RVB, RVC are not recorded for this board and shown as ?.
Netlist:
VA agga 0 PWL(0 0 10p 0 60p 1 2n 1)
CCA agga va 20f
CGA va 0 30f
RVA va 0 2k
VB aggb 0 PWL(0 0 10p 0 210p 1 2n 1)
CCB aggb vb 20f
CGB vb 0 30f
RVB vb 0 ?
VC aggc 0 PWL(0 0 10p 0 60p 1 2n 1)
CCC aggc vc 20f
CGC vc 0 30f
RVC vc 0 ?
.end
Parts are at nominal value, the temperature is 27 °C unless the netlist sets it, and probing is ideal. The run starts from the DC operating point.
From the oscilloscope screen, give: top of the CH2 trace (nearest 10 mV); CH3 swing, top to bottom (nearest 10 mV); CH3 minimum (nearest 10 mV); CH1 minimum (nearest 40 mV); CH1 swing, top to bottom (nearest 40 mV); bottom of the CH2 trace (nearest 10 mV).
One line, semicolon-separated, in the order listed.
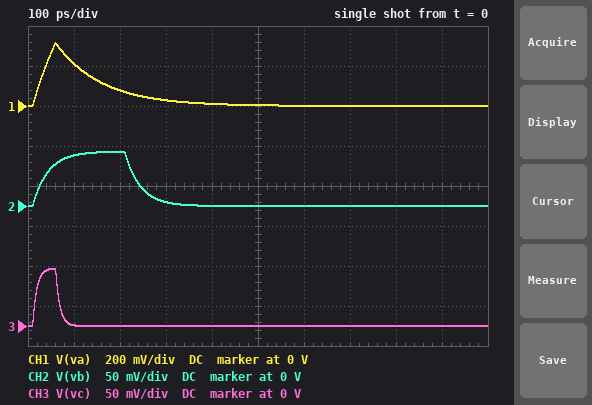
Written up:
70 mV; 70 mV; 0 V; 0 V; 320 mV; 0 V
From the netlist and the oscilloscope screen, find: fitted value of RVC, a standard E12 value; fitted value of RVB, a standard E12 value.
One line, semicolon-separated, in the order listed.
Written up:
180 Ω; 680 Ω
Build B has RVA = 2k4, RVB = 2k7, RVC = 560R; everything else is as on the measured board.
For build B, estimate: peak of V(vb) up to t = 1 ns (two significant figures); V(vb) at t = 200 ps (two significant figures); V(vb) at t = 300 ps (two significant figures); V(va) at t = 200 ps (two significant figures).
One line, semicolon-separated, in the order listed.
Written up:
210 mV; 200 mV; 110 mV; 100 mV
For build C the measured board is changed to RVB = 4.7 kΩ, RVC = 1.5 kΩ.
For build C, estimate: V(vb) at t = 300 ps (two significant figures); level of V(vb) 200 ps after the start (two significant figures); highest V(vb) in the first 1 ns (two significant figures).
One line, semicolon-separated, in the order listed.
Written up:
180 mV; 260 mV; 270 mV
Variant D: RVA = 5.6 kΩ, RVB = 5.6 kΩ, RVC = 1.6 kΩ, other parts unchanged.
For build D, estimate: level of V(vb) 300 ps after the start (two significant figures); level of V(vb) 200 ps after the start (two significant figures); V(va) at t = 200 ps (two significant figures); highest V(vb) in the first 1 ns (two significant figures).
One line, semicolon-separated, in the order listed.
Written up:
210 mV; 280 mV; 220 mV; 290 mV
